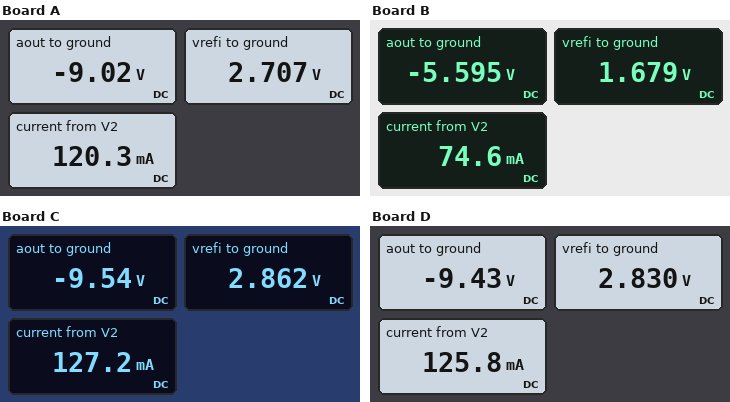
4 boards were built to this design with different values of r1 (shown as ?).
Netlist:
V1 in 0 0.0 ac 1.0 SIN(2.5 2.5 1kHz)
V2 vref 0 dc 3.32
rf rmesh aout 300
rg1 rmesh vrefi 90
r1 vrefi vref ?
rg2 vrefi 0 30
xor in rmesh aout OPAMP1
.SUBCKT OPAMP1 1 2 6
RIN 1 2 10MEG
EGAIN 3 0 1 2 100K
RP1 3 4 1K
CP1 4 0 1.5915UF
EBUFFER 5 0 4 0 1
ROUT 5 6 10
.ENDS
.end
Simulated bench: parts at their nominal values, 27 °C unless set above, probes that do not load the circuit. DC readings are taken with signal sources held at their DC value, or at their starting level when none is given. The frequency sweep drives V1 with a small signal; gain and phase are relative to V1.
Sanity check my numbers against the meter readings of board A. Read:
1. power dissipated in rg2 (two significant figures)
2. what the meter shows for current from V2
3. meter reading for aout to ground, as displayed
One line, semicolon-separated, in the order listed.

240 mW; 120.3 mA; -9.02 V
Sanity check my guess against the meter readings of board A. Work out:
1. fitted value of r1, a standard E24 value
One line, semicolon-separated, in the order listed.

5.1 Ω
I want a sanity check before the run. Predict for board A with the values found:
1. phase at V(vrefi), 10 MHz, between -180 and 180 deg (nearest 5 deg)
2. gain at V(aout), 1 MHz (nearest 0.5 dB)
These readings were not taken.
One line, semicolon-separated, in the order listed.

-75 deg; 11.5 dB
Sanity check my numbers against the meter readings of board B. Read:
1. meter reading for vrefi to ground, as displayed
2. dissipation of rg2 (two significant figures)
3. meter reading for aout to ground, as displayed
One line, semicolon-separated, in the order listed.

1.679 V; 94 mW; -5.595 V
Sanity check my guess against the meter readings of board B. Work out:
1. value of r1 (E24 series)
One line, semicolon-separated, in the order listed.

22 Ω
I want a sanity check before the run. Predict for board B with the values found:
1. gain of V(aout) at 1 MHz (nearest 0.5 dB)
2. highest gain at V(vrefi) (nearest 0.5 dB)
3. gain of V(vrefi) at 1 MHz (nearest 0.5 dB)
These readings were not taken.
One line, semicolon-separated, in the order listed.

11.0 dB; -18.0 dB; -19.0 dB
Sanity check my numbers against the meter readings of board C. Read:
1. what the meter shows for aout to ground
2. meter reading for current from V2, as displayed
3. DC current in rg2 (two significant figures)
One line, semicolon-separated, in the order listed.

-9.54 V; 127.2 mA; 95 mA
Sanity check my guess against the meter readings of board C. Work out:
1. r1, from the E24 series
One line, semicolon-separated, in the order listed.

3.6 Ω
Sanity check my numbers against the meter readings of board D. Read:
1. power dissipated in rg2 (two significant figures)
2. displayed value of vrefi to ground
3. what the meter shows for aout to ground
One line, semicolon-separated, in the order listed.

270 mW; 2.830 V; -9.43 V
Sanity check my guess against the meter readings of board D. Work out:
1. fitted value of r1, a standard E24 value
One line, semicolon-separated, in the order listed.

3.9 Ω
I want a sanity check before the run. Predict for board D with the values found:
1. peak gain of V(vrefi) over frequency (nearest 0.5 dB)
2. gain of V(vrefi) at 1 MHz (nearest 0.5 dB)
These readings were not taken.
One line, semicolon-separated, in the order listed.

-28.5 dB; -29.5 dB
